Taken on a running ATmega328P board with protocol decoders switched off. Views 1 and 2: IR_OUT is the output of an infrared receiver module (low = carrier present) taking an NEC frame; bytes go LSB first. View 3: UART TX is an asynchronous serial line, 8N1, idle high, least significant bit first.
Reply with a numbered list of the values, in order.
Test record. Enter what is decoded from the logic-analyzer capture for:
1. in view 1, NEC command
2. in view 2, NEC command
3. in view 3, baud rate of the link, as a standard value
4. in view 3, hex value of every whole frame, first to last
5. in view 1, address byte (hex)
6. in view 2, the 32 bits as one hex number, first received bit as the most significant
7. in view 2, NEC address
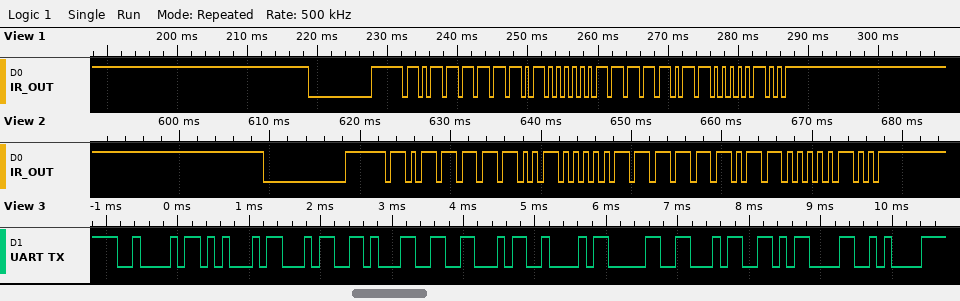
1. 0xDF
2. 0xDF
3. 9600 baud
4. 42 45 34 31 46 42 30 34 0D 0A
5. 0xFD
6. 0xBE41FB04
7. 0x7D
